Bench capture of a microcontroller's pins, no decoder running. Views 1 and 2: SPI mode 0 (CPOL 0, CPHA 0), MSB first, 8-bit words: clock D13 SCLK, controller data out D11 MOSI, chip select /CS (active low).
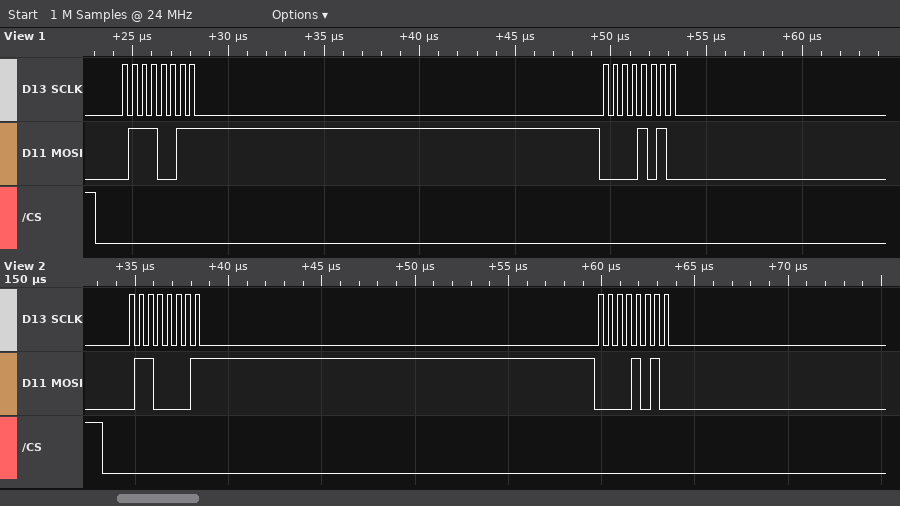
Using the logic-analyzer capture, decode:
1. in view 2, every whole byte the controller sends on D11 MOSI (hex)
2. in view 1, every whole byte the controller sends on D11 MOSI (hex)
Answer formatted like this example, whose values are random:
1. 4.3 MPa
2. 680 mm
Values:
1. 0x61 0x0A
2. 73 0A
